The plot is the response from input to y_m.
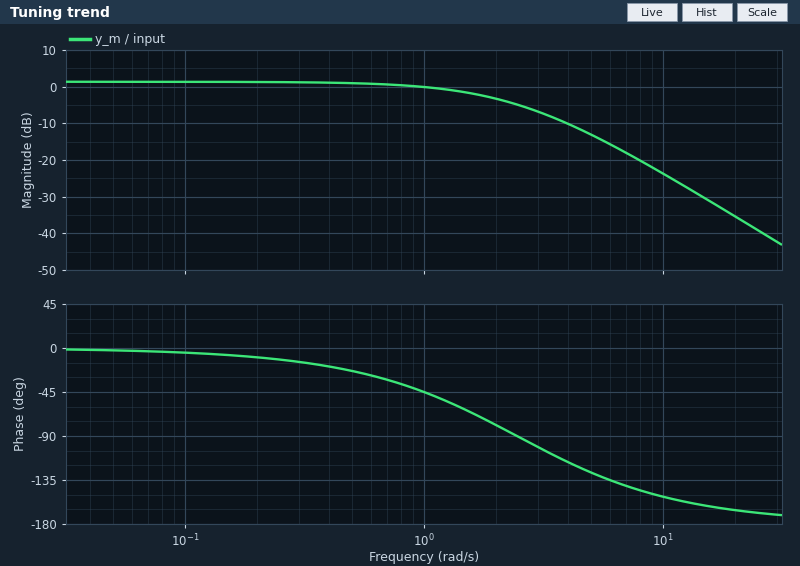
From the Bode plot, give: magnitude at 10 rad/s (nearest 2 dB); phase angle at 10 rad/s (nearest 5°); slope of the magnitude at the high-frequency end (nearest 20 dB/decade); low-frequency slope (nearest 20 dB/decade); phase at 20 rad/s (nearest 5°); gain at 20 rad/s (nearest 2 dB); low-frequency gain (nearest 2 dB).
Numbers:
-24 dB
-150°
-40 dB/decade
0 dB/decade
-165°
-36 dB
2 dB
